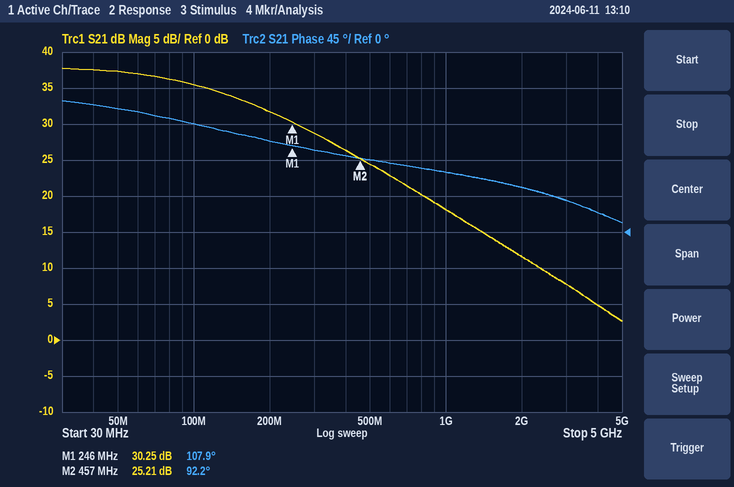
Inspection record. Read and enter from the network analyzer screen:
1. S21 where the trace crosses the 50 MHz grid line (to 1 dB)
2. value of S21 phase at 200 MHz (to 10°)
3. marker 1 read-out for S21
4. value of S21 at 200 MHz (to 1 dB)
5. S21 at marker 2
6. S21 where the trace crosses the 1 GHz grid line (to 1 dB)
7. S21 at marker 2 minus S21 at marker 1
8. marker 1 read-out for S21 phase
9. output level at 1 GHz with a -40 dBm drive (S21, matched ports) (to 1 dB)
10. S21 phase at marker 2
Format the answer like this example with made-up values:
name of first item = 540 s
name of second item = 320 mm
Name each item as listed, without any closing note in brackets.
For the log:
S21 where the trace crosses the 50 MHz grid line = 37 dB
value of S21 phase at 200 MHz = 110°
marker 1 read-out for S21 = 30.25 dB
value of S21 at 200 MHz = 32 dB
S21 at marker 2 = 25.21 dB
S21 where the trace crosses the 1 GHz grid line = 18 dB
S21 at marker 2 minus S21 at marker 1 = -5.04 dB
marker 1 read-out for S21 phase = 107.9°
output level at 1 GHz with a -40 dBm drive (S21, matched ports) = -22 dBm
S21 phase at marker 2 = 92.2°
